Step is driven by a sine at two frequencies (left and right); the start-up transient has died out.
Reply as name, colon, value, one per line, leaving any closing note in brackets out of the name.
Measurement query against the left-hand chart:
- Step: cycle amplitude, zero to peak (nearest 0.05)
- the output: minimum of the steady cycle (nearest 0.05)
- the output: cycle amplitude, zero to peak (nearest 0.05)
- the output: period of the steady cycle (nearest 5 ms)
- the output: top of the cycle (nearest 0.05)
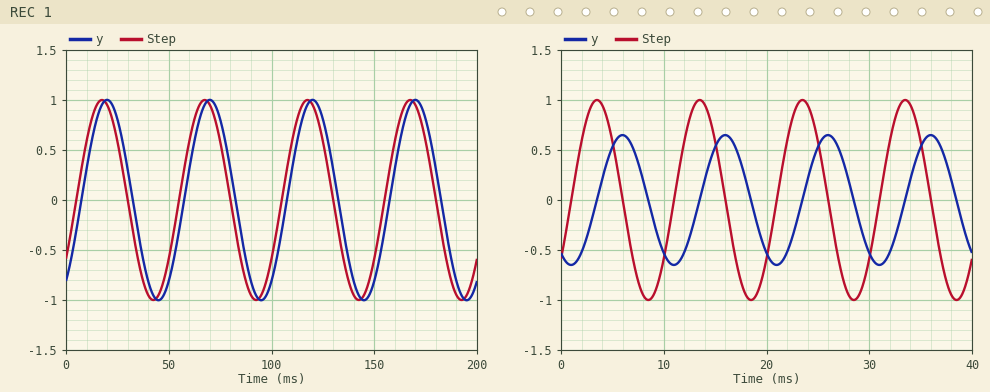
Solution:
Step: cycle amplitude, zero to peak: 1.00
the output: minimum of the steady cycle: -1.00
the output: cycle amplitude, zero to peak: 1.00
the output: period of the steady cycle: 50 ms
the output: top of the cycle: 1.00
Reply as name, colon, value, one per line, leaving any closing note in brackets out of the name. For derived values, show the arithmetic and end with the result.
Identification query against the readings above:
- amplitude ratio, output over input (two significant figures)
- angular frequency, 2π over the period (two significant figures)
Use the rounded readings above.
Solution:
amplitude ratio, output over input: 1 / 1 = 1.0
angular frequency, 2π over the period: 2π / 50 = 0.13 rad/ms
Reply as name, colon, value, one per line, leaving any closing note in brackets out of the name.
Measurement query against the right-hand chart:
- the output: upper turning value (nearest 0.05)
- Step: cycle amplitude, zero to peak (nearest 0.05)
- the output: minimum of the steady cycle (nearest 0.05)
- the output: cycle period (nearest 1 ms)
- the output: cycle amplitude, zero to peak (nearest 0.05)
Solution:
the output: upper turning value: 0.65
Step: cycle amplitude, zero to peak: 1.00
the output: minimum of the steady cycle: -0.65
the output: cycle period: 10 ms
the output: cycle amplitude, zero to peak: 0.65
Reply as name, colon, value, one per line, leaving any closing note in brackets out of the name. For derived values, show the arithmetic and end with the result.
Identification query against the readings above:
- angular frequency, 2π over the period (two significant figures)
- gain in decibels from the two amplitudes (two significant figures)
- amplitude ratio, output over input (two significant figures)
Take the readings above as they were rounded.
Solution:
angular frequency, 2π over the period: 2π / 10 = 0.63 rad/ms
gain in decibels from the two amplitudes: 20 log10(0.65 / 1) = -3.7 dB
amplitude ratio, output over input: 0.65 / 1 = 0.65
